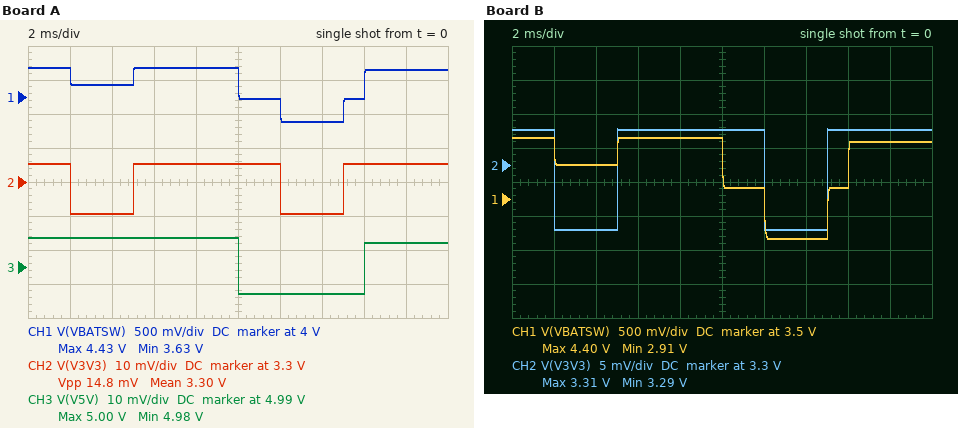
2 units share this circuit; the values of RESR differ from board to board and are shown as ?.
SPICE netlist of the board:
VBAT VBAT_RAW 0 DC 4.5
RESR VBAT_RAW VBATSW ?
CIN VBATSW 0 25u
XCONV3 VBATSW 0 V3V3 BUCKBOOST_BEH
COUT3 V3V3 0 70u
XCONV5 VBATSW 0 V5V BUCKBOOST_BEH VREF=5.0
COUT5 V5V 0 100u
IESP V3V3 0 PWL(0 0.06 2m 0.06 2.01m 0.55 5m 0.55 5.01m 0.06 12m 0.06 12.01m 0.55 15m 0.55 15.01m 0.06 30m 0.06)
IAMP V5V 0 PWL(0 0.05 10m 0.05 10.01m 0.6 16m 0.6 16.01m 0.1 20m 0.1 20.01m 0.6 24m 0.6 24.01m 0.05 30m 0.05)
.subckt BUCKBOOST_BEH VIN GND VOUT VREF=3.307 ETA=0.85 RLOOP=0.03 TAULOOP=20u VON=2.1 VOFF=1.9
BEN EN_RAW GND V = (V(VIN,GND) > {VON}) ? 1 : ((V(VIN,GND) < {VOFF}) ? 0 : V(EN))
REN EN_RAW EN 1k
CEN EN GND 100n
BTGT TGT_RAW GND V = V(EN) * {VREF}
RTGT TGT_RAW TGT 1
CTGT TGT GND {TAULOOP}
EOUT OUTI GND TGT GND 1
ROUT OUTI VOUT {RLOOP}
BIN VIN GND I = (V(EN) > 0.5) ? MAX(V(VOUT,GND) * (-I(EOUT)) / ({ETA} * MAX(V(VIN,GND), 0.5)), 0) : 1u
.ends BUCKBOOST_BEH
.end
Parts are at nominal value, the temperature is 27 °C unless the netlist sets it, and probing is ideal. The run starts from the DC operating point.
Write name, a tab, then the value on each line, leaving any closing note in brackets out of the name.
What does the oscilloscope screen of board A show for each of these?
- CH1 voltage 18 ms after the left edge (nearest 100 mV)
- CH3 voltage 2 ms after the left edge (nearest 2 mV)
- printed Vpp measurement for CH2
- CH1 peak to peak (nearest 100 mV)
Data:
CH1 voltage 18 ms after the left edge	4.4 V
CH3 voltage 2 ms after the left edge	4.998 V
printed Vpp measurement for CH2	14.8 mV
CH1 peak to peak	800 mV
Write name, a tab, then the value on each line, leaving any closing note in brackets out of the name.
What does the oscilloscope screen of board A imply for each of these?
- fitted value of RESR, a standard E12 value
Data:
fitted value of RESR, a standard E12 value	0.56 Ω
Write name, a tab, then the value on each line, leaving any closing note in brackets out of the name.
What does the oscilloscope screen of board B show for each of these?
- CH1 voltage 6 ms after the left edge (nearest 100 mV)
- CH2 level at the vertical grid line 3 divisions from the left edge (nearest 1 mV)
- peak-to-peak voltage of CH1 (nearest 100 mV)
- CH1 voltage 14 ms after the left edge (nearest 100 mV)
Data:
CH1 voltage 6 ms after the left edge	4.4 V
CH2 level at the vertical grid line 3 divisions from the left edge	3.305 V
peak-to-peak voltage of CH1	1.5 V
CH1 voltage 14 ms after the left edge	2.9 V
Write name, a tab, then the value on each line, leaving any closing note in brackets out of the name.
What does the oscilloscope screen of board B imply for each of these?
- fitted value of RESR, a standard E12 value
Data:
fitted value of RESR, a standard E12 value	0.82 Ω
